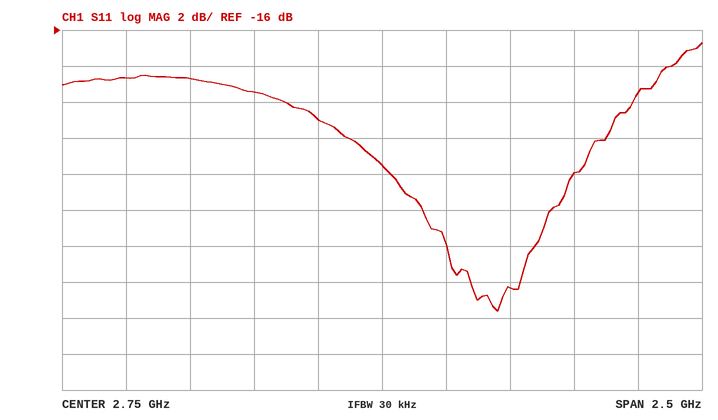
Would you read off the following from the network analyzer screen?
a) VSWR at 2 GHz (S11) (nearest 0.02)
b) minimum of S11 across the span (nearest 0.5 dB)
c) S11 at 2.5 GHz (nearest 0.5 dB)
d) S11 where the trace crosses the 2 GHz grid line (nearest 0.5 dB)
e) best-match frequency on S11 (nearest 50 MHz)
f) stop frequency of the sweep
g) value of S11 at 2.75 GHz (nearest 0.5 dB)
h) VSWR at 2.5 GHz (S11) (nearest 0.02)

1.26
-31.5 dB
-21.0 dB
-18.5 dB
3.20 GHz
4 GHz
-23.5 dB
1.20
